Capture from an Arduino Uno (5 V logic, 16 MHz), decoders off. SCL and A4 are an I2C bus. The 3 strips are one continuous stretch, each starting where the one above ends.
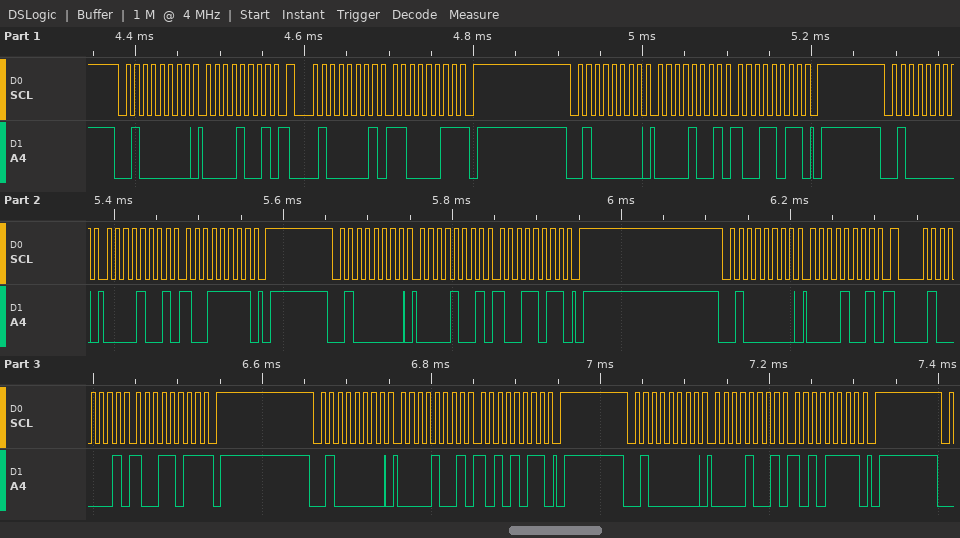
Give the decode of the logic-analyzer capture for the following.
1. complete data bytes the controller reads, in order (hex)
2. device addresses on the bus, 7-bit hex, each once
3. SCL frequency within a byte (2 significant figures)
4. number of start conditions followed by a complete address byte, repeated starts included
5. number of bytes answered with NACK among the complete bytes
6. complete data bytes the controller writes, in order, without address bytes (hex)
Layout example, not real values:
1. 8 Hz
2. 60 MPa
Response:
1. C3 9B
2. 0x20
3. 100 kHz
4. 9
5. 2
6. 09 09 9B 09 9F 09 9B 09 09 AB 09 AF
